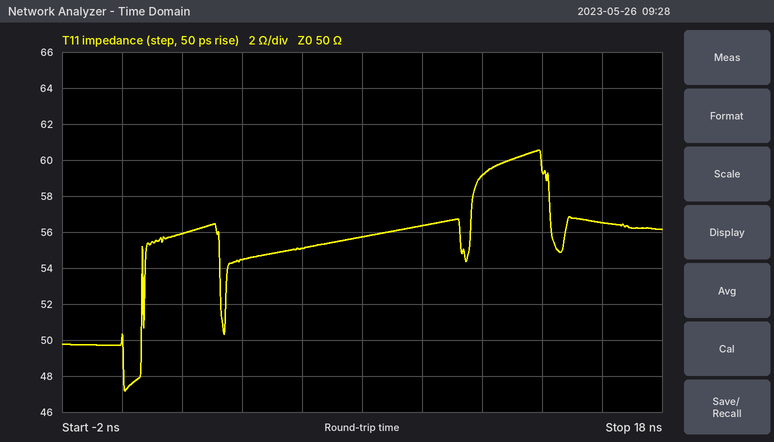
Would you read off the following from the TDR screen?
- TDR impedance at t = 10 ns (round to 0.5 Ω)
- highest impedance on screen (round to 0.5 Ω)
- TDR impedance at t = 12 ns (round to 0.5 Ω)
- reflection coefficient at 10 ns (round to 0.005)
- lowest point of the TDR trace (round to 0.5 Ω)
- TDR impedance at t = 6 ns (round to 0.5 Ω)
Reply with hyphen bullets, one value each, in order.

- 56.5 Ω
- 60.5 Ω
- 59.0 Ω
- +0.060
- 47.0 Ω
- 55.0 Ω
